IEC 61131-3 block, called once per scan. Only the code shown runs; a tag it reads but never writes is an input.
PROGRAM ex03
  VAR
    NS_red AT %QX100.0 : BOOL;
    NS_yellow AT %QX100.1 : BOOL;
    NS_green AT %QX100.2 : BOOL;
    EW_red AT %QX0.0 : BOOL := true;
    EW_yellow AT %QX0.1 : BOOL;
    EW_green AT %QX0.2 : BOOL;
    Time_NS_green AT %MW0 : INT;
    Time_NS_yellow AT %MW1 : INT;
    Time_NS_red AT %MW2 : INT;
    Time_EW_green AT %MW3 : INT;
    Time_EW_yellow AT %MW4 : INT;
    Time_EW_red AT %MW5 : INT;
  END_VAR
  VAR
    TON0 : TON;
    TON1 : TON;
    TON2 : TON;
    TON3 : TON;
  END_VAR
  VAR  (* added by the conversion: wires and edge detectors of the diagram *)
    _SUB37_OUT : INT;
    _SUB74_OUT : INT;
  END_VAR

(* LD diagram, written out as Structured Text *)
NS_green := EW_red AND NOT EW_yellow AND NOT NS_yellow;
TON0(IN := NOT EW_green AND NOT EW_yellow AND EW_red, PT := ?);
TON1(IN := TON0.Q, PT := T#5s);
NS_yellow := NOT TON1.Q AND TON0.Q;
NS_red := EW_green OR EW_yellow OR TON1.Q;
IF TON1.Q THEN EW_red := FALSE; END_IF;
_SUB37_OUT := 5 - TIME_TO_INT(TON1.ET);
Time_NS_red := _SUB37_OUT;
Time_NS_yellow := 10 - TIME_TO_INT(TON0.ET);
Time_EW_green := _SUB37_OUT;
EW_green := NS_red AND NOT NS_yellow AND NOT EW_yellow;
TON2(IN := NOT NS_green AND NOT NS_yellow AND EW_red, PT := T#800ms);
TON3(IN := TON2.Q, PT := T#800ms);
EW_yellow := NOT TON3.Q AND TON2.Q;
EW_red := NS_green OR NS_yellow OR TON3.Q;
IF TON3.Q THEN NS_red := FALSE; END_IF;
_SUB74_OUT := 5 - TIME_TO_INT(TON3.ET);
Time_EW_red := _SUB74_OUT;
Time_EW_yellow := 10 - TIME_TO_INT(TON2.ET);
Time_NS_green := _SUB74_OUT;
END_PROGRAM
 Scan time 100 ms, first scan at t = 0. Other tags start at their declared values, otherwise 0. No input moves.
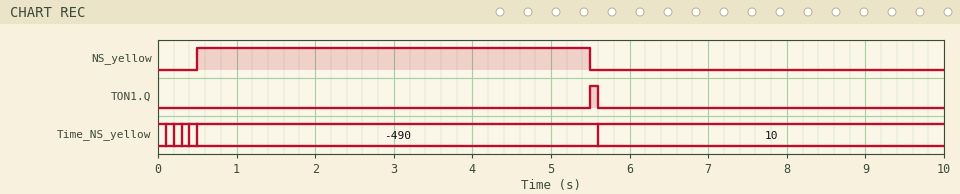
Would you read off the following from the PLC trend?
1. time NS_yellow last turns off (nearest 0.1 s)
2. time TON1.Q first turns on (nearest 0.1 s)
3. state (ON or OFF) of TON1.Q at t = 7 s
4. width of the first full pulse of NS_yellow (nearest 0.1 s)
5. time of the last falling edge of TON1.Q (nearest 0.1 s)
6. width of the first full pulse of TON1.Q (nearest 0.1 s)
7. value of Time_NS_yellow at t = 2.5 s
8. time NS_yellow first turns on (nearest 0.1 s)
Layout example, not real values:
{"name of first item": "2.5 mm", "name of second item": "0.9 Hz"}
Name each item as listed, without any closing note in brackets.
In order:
{"time NS_yellow last turns off": "5.5 s", "time TON1.Q first turns on": "5.5 s", "state (ON or OFF) of TON1.Q at t = 7 s": "OFF", "width of the first full pulse of NS_yellow": "5.0 s", "time of the last falling edge of TON1.Q": "5.6 s", "width of the first full pulse of TON1.Q": "0.1 s", "value of Time_NS_yellow at t = 2.5 s": "-490", "time NS_yellow first turns on": "0.5 s"}
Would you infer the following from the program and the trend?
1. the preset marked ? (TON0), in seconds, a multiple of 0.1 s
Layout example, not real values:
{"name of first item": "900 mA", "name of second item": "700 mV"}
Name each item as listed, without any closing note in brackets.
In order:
{"the preset marked ? (TON0), in seconds, a multiple of 0.1 s": "0.5 s"}
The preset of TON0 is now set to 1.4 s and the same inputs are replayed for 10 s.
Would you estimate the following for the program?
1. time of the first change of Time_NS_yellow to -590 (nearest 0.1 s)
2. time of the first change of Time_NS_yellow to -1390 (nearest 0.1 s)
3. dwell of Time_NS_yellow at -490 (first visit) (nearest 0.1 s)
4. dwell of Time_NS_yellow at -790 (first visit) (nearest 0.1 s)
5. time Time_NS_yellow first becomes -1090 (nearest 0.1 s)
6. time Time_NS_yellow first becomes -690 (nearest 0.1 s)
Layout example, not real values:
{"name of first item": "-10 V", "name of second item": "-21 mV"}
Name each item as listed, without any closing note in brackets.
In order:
{"time of the first change of Time_NS_yellow to -590": "0.6 s", "time of the first change of Time_NS_yellow to -1390": "1.4 s", "dwell of Time_NS_yellow at -490 (first visit)": "0.1 s", "dwell of Time_NS_yellow at -790 (first visit)": "0.1 s", "time Time_NS_yellow first becomes -1090": "1.1 s", "time Time_NS_yellow first becomes -690": "0.7 s"}
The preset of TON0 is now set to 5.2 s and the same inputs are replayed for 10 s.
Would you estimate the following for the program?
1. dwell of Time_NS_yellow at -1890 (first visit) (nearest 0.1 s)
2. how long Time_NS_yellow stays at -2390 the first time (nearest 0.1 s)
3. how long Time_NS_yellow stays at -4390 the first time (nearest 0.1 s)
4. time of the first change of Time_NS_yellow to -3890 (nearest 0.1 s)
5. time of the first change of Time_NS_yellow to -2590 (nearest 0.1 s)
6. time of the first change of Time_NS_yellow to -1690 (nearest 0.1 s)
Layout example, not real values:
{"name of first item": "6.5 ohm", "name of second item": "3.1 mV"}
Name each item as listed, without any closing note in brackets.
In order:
{"dwell of Time_NS_yellow at -1890 (first visit)": "0.1 s", "how long Time_NS_yellow stays at -2390 the first time": "0.1 s", "how long Time_NS_yellow stays at -4390 the first time": "0.1 s", "time of the first change of Time_NS_yellow to -3890": "3.9 s", "time of the first change of Time_NS_yellow to -2590": "2.6 s", "time of the first change of Time_NS_yellow to -1690": "1.7 s"}
